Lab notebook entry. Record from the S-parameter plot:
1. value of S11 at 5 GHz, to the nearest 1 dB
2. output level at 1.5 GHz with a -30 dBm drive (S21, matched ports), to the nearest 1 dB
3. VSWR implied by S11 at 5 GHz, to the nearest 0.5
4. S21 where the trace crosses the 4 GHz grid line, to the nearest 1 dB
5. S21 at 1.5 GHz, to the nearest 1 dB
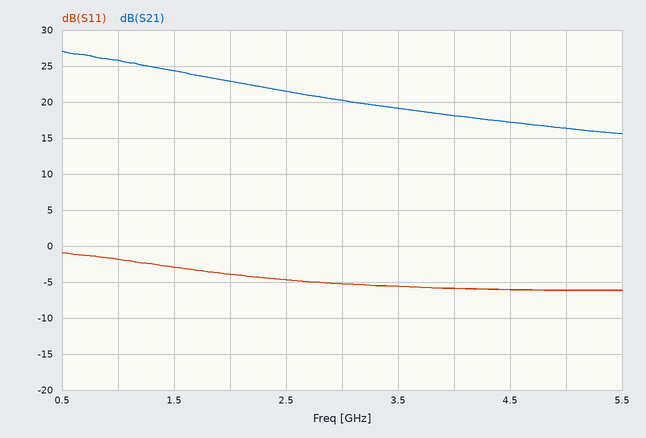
-6 dB
-6 dBm
3.0
18 dB
24 dB
